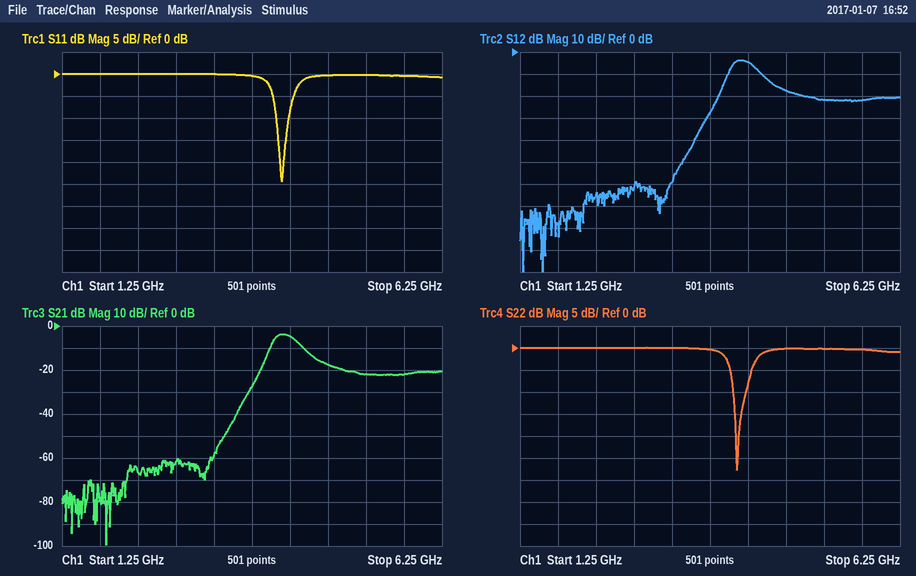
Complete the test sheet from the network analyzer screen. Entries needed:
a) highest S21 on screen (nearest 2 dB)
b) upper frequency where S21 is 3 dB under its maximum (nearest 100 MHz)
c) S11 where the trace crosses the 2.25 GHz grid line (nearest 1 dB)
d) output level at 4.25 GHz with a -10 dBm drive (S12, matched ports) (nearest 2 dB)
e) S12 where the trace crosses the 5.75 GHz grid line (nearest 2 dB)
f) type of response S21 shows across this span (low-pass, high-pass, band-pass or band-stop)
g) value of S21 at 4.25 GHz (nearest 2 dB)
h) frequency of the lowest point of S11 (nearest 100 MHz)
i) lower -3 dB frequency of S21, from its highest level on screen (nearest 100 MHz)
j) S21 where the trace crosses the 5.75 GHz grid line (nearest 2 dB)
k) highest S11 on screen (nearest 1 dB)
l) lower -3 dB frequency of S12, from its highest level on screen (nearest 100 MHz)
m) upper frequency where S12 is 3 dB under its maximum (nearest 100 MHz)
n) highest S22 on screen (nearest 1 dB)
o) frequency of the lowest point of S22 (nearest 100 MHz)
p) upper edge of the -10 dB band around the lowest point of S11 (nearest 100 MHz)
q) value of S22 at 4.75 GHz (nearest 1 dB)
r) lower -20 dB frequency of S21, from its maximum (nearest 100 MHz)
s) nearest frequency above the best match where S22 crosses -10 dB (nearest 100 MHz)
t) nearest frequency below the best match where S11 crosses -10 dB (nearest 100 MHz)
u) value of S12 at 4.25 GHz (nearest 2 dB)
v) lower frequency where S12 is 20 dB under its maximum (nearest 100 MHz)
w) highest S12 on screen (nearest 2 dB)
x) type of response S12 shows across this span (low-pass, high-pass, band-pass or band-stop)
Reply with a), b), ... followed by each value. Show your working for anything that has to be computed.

a) -4 dB
b) 4.3 GHz
c) 0 dB
d) -10 dBm + (-4 dB) = -14 dBm
e) -22 dB
f) band-pass
g) -4 dB
h) 4.1 GHz
i) 4.0 GHz
j) -22 dB
k) 0 dB
l) 4.0 GHz
m) 4.3 GHz
n) 0 dB
o) 4.1 GHz
p) 4.2 GHz
q) 0 dB
r) 3.8 GHz
s) 4.2 GHz
t) 4.1 GHz
u) -4 dB
v) 3.8 GHz
w) -4 dB
x) band-pass
